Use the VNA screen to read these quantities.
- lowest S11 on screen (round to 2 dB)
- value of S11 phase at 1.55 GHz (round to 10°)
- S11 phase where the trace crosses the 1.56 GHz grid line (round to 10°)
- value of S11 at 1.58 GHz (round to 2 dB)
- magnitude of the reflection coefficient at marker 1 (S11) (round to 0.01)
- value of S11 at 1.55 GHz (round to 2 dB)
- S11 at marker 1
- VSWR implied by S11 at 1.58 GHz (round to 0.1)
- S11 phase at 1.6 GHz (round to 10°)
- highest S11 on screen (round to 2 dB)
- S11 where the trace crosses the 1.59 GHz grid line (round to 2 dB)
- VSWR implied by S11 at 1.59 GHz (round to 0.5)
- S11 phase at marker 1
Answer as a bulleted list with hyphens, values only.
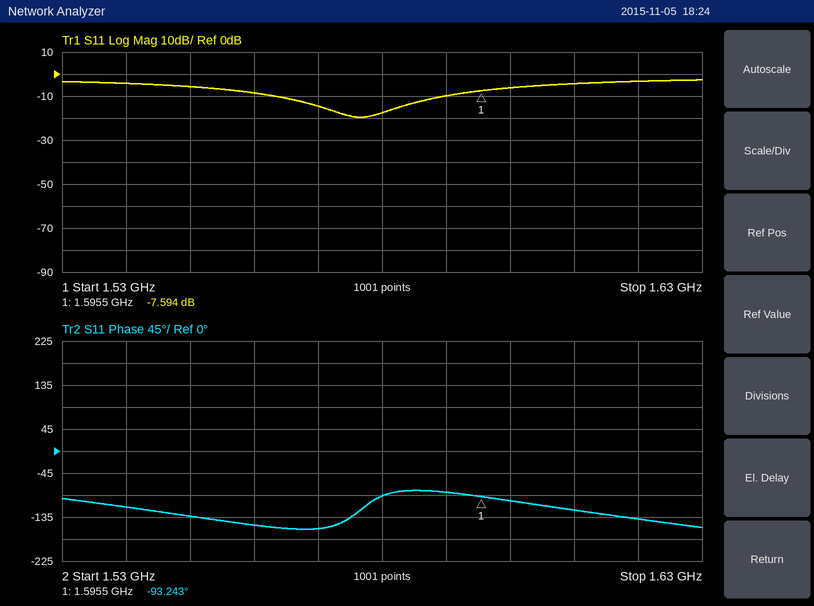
- -20 dB
- -130°
- -150°
- -18 dB
- 0.42
- -6 dB
- -7.594 dB
- 1.3
- -100°
- -2 dB
- -10 dB
- 2.0
- -93.243°
